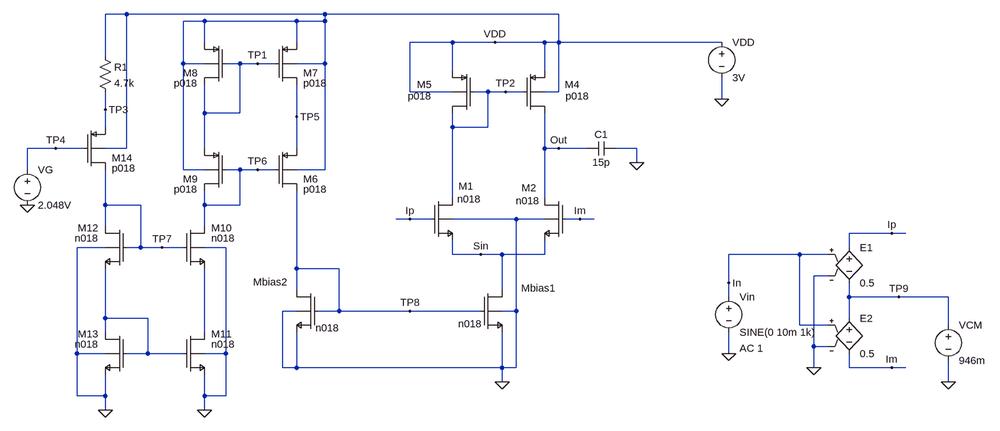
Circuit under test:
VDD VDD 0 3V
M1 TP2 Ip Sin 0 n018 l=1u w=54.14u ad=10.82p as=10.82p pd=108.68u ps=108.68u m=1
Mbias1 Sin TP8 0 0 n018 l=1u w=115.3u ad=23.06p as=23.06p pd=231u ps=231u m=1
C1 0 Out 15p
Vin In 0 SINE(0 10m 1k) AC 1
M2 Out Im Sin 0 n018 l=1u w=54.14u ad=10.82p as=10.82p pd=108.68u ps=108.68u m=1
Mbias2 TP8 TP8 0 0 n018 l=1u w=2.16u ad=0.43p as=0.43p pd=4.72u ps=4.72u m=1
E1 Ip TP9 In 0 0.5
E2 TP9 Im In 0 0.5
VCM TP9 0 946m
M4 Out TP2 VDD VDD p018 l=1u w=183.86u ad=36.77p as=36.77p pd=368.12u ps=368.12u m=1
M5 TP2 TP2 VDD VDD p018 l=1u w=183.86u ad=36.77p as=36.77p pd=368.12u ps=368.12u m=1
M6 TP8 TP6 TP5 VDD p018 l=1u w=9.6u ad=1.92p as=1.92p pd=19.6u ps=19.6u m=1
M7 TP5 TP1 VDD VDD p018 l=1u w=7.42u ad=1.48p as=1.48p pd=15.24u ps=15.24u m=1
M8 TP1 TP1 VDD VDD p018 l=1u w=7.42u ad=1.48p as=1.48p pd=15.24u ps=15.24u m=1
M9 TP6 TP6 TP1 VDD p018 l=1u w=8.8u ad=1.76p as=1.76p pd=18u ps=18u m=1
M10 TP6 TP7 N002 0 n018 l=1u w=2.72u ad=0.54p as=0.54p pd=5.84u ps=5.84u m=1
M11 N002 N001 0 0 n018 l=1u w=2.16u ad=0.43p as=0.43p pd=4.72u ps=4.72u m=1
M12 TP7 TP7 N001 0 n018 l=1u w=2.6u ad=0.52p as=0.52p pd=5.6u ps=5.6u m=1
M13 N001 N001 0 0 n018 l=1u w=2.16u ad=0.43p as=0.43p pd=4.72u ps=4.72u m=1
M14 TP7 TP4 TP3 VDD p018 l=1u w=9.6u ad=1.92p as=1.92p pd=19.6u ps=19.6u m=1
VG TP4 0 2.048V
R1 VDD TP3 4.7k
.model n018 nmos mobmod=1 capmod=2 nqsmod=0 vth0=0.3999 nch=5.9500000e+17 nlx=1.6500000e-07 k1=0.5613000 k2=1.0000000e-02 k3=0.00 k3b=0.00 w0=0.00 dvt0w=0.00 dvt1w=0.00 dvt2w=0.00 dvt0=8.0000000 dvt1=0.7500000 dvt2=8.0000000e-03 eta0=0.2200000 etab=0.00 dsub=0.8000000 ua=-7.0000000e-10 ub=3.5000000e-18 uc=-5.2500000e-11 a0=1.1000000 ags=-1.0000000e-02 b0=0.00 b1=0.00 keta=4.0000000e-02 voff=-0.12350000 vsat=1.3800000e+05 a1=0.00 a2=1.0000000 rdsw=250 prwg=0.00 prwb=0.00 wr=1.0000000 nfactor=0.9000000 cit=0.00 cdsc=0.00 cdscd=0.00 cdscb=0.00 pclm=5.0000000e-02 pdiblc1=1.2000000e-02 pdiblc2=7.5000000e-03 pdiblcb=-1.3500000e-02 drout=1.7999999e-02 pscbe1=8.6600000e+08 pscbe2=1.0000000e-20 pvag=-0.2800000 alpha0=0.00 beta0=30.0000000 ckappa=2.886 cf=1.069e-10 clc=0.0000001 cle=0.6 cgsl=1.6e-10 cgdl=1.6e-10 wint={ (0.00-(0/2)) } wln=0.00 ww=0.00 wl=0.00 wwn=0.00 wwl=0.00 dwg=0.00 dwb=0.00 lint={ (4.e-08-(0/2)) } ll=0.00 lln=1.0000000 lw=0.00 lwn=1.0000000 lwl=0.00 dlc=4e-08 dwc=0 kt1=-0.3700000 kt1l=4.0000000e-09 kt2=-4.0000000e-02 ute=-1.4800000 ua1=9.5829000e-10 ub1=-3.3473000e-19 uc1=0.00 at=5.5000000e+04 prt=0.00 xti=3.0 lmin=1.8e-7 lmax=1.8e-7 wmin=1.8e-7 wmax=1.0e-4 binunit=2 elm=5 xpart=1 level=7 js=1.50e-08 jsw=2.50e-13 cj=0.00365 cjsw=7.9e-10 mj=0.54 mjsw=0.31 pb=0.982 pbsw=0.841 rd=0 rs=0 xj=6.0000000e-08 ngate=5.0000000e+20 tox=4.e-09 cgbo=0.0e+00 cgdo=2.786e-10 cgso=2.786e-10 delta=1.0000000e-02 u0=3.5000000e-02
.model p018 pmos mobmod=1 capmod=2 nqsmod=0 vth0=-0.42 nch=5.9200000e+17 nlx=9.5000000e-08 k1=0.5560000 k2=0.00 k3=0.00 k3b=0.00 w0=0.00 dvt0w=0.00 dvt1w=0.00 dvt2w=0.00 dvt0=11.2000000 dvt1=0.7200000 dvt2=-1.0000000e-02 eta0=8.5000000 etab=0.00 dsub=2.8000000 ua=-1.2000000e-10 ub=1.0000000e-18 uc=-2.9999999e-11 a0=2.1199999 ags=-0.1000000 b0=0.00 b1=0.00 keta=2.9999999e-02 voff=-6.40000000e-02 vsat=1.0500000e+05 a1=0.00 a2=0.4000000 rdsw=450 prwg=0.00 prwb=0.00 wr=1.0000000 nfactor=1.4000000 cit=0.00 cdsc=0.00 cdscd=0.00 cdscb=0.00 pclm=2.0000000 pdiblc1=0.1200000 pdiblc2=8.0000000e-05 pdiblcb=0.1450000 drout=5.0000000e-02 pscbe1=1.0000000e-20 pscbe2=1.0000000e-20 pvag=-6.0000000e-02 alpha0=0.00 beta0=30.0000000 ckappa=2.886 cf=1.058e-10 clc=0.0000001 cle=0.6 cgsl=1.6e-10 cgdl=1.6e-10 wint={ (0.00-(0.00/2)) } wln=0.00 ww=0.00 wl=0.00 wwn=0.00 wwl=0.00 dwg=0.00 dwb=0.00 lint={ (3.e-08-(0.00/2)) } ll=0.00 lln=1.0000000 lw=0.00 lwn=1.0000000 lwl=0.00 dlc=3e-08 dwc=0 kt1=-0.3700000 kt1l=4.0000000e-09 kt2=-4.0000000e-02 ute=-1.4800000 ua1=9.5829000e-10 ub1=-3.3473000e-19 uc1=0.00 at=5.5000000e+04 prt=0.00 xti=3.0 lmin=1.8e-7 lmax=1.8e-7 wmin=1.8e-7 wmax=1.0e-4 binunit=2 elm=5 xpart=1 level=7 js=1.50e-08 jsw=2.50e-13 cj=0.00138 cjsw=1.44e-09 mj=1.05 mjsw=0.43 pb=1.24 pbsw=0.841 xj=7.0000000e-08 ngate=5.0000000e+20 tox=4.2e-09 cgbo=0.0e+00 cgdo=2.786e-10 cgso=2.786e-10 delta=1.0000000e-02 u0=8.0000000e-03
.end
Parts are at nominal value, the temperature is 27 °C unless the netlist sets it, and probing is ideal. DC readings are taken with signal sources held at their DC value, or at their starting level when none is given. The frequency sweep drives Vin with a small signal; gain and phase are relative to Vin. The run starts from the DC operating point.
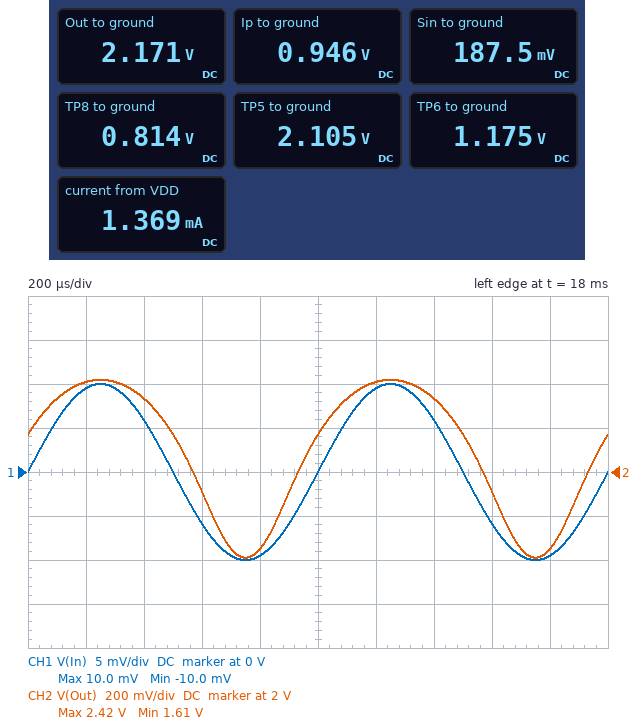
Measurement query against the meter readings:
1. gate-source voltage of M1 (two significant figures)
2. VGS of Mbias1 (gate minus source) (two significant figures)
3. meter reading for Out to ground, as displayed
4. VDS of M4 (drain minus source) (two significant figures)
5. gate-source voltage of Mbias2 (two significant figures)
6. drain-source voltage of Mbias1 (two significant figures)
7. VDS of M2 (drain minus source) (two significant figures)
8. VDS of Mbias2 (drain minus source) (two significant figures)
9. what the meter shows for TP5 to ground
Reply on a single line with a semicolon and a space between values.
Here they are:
760 mV; 810 mV; 2.171 V; -830 mV; 810 mV; 190 mV; 2.0 V; 810 mV; 2.105 V
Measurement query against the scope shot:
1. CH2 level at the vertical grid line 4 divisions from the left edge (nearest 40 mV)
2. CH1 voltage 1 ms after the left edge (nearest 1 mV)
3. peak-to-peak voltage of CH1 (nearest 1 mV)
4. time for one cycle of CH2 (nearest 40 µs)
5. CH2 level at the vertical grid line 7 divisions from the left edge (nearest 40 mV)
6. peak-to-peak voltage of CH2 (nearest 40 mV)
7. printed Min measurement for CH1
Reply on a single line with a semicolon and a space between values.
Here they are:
1.64 V; 0 V; 20 mV; 1.00 ms; 2.32 V; 800 mV; -10.0 mV
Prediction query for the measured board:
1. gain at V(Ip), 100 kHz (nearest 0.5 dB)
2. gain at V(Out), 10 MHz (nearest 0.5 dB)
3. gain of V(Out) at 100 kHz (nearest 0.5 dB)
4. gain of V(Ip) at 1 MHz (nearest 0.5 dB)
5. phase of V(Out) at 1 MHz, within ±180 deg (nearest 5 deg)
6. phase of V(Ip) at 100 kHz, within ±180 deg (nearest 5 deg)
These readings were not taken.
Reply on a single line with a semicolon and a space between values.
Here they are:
-6.0 dB; 9.0 dB; 30.5 dB; -6.0 dB; -50 deg; 0 deg
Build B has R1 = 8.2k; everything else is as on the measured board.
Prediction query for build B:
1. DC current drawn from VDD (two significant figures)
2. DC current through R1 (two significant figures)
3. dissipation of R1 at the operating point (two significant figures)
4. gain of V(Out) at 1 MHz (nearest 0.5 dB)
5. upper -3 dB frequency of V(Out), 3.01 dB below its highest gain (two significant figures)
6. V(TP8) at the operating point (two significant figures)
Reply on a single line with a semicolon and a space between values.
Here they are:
1.2 mA; 21 µA; 3.7 µW; 26.5 dB; 820 kHz; 760 mV
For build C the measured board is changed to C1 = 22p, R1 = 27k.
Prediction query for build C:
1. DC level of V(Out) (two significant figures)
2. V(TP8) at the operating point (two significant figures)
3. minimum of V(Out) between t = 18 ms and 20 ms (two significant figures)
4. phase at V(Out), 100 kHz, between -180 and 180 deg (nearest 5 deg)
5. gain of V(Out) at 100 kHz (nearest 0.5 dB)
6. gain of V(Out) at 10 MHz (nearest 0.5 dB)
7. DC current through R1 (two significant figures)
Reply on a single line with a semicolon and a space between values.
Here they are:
2.3 V; 640 mV; 1.7 V; -10 deg; 31.0 dB; 4.5 dB; 10 µA
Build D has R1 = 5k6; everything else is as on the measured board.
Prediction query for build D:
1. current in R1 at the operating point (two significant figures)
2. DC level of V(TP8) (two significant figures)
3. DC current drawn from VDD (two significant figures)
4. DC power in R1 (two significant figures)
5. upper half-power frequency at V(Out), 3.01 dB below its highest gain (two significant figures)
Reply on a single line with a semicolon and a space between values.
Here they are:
25 µA; 800 mV; 1.3 mA; 3.6 µW; 840 kHz
